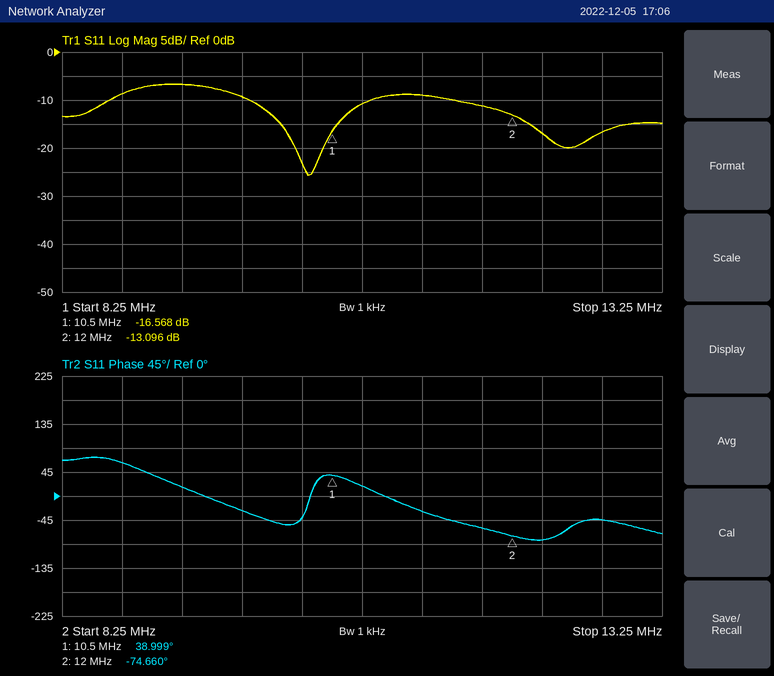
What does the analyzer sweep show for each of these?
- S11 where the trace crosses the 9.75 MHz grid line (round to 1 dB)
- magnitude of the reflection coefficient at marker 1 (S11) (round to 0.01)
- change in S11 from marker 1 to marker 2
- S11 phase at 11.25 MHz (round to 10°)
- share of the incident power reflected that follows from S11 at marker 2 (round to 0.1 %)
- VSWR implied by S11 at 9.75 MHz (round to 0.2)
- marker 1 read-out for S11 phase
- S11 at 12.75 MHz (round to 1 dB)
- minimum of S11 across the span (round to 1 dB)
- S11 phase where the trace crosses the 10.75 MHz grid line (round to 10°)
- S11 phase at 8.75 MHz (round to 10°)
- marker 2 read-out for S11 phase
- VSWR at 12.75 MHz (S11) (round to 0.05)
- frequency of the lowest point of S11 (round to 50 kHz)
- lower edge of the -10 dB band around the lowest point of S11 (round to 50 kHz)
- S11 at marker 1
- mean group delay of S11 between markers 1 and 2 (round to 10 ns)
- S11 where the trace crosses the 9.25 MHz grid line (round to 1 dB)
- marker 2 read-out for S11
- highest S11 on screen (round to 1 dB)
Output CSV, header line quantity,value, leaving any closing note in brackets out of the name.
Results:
quantity,value
S11 where the trace crosses the 9.75 MHz grid line,-9 dB
magnitude of the reflection coefficient at marker 1 (S11),0.15
change in S11 from marker 1 to marker 2,3.472 dB
S11 phase at 11.25 MHz,-30°
share of the incident power reflected that follows from S11 at marker 2,4.9 %
VSWR implied by S11 at 9.75 MHz,2.0
marker 1 read-out for S11 phase,38.999°
S11 at 12.75 MHz,-17 dB
minimum of S11 across the span,-26 dB
S11 phase where the trace crosses the 10.75 MHz grid line,20°
S11 phase at 8.75 MHz,60°
marker 2 read-out for S11 phase,-74.660°
VSWR at 12.75 MHz (S11),1.35
frequency of the lowest point of S11,10.30 MHz
lower edge of the -10 dB band around the lowest point of S11,9.80 MHz
S11 at marker 1,-16.568 dB
mean group delay of S11 between markers 1 and 2,210 ns
S11 where the trace crosses the 9.25 MHz grid line,-7 dB
marker 2 read-out for S11,-13.096 dB
highest S11 on screen,-7 dB
